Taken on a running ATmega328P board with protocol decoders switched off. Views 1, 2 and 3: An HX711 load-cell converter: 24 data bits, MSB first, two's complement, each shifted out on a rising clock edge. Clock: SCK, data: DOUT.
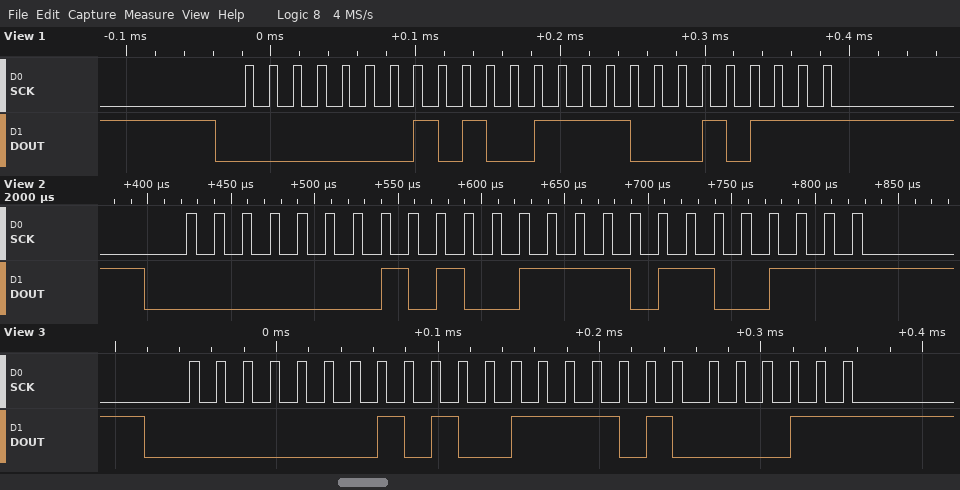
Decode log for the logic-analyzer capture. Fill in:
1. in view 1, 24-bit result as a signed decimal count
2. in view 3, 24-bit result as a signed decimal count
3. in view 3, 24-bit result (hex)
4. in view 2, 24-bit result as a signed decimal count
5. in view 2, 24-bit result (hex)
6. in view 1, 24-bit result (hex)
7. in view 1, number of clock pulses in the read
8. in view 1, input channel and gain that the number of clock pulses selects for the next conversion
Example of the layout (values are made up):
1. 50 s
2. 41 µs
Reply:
1. 85783
2. 85827
3. 0x014F43
4. 85863
5. 0x014F67
6. 0x014F17
7. 25
8. channel A, gain 128
